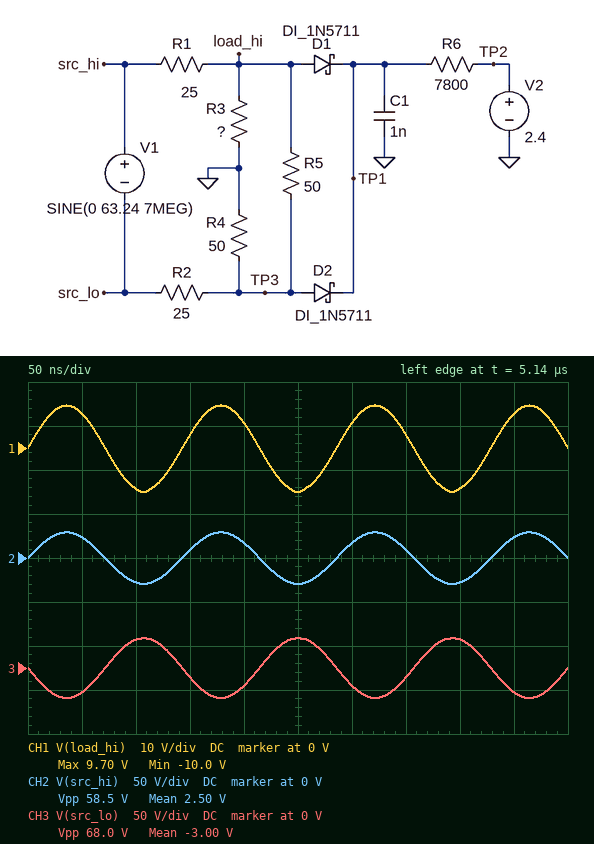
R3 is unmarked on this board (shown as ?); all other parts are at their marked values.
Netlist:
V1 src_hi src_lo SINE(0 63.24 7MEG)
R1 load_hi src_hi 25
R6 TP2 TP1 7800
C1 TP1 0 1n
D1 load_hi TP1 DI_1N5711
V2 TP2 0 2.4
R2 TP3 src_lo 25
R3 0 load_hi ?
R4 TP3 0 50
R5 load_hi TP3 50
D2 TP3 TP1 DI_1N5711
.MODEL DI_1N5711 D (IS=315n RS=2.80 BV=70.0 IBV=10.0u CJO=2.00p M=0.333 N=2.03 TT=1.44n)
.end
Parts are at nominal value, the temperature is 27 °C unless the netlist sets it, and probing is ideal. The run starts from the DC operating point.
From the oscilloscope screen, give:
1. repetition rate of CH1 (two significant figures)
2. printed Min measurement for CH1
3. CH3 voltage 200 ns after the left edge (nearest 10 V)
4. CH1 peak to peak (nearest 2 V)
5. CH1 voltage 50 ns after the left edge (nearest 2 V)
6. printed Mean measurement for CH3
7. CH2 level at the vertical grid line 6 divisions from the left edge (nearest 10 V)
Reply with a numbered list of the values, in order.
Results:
1. 7.0 MHz
2. -10.0 V
3. -20 V
4. 20 V
5. 8 V
6. -3.00 V
7. 20 V
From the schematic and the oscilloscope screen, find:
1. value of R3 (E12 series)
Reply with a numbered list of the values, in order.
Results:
1. 33 Ω
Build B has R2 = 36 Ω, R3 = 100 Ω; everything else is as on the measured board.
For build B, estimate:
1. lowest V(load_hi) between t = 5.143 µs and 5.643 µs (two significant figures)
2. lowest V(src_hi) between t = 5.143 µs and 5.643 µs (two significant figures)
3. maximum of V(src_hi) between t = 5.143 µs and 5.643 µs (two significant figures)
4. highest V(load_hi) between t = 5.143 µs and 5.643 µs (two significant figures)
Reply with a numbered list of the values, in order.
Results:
1. -16 V
2. -32 V
3. 31 V
4. 15 V
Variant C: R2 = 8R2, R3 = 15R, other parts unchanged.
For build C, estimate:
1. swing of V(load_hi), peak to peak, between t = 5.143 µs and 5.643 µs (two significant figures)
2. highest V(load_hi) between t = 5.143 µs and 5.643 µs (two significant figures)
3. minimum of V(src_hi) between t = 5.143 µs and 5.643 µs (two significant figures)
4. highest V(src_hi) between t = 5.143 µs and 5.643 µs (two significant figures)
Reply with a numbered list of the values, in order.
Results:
1. 14 V
2. 6.7 V
3. -33 V
4. 32 V
